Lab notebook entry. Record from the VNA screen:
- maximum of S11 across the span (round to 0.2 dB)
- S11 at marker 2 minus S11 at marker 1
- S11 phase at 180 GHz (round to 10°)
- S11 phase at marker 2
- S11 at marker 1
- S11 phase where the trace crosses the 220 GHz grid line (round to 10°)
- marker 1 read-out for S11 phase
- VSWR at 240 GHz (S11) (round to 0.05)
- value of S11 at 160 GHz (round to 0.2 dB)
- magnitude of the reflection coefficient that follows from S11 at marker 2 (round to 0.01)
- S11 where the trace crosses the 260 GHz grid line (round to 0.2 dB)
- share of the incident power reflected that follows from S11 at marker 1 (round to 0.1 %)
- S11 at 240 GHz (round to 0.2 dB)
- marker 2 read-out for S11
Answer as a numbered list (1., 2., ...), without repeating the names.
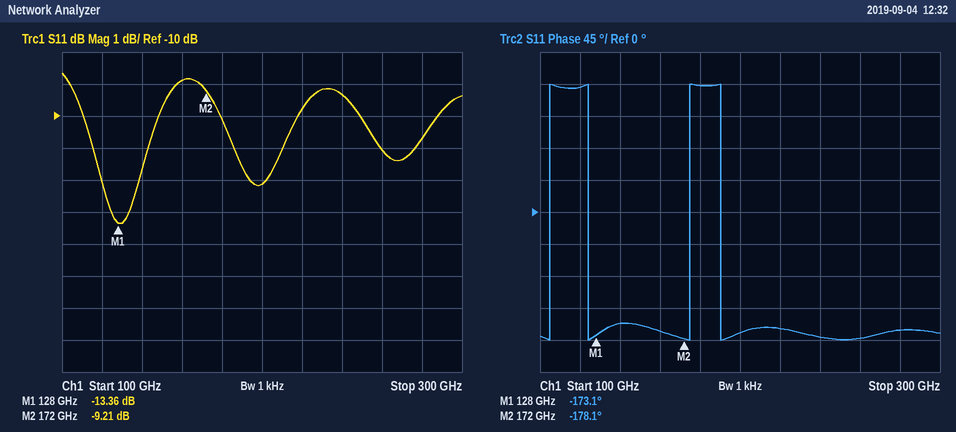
1. -8.6 dB
2. 4.15 dB
3. 180°
4. -178.1°
5. -13.36 dB
6. -160°
7. -173.1°
8. 2.05
9. -8.8 dB
10. 0.35
11. -11.0 dB
12. 4.6 %
13. -9.4 dB
14. -9.21 dB
